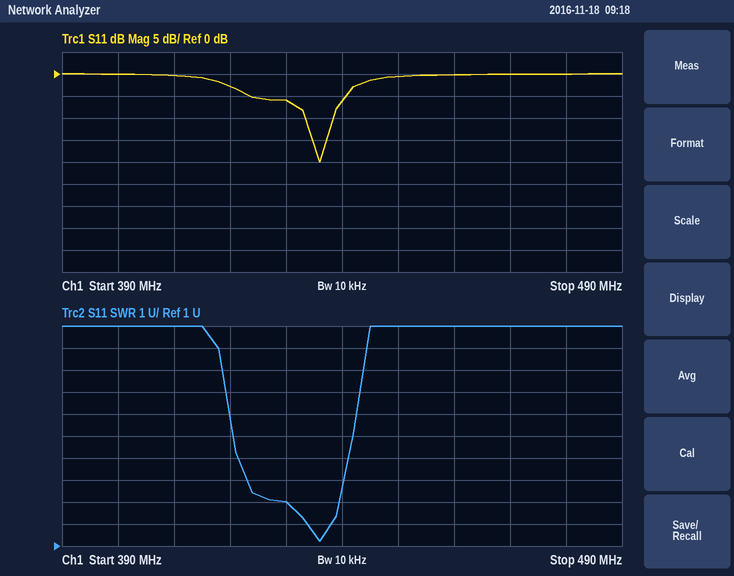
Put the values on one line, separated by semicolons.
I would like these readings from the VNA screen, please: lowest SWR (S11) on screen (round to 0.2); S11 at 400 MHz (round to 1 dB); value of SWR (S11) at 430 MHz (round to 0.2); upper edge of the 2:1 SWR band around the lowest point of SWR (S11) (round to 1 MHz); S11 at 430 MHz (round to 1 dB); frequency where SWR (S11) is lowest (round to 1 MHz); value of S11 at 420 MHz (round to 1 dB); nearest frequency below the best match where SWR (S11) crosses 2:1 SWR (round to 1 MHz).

1.2; 0 dB; 3.0; 438 MHz; -6 dB; 436 MHz; -3 dB; 434 MHz
